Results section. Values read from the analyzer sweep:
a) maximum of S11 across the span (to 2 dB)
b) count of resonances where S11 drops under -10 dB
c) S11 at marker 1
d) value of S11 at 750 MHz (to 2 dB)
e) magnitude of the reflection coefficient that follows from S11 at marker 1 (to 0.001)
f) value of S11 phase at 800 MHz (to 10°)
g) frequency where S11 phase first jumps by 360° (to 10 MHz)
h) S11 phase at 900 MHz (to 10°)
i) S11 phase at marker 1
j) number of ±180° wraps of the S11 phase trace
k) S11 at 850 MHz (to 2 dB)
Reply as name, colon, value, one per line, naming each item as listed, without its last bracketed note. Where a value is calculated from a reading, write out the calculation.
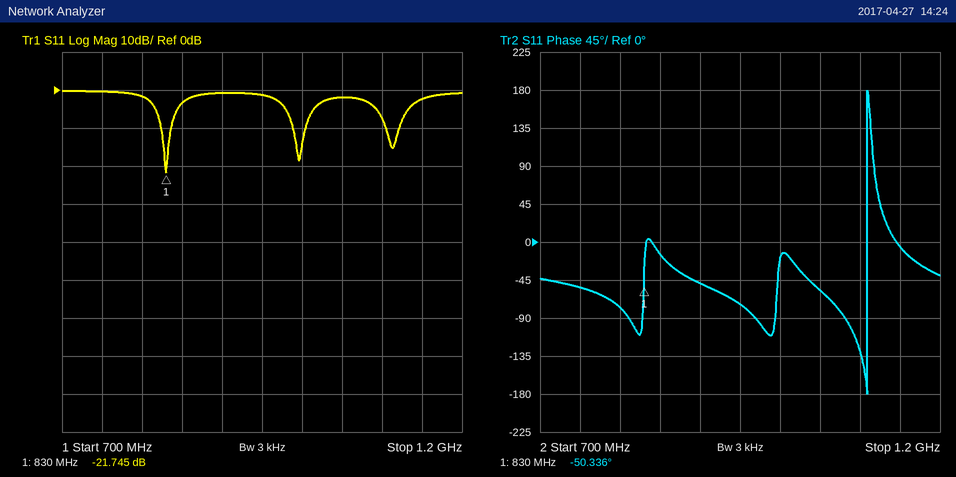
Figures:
maximum of S11 across the span: 0 dB
count of resonances where S11 drops under -10 dB: 3
S11 at marker 1: -21.745 dB
value of S11 at 750 MHz: 0 dB
magnitude of the reflection coefficient that follows from S11 at marker 1: 10^(-21.745/20) ≈ 0.082
value of S11 phase at 800 MHz: -80°
frequency where S11 phase first jumps by 360°: 1.11 GHz
S11 phase at 900 MHz: -50°
S11 phase at marker 1: -50.336°
number of ±180° wraps of the S11 phase trace: 1
S11 at 850 MHz: -4 dB
